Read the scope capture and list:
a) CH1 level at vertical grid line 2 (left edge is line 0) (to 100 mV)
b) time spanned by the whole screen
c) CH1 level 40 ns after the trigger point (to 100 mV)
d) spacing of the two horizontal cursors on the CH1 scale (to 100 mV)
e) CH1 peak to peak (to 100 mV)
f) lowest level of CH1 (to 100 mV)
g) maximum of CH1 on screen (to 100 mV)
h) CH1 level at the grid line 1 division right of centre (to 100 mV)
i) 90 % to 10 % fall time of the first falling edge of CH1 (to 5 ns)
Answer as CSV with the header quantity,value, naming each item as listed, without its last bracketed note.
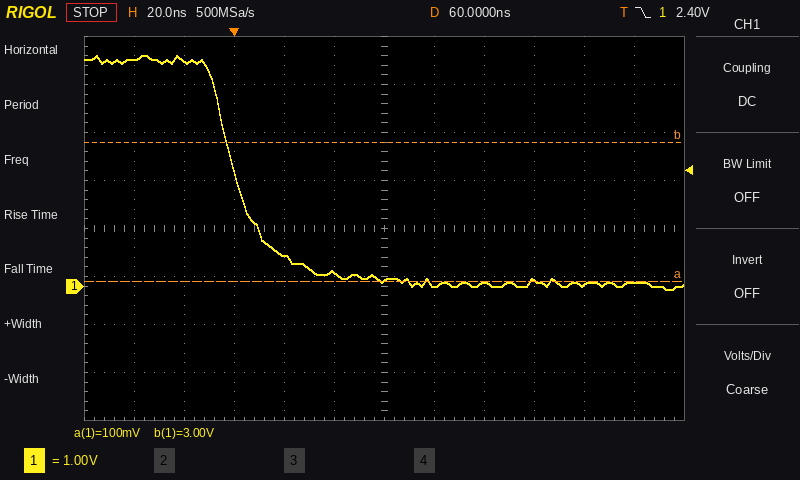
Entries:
quantity,value
CH1 level at vertical grid line 2 (left edge is line 0),4.7 V
time spanned by the whole screen,240 ns
CH1 level 40 ns after the trigger point,300 mV
spacing of the two horizontal cursors on the CH1 scale,2.9 V
CH1 peak to peak,4.9 V
lowest level of CH1,-100 mV
maximum of CH1 on screen,4.8 V
CH1 level at the grid line 1 division right of centre,0.0 V
90 % to 10 % fall time of the first falling edge of CH1,30 ns
